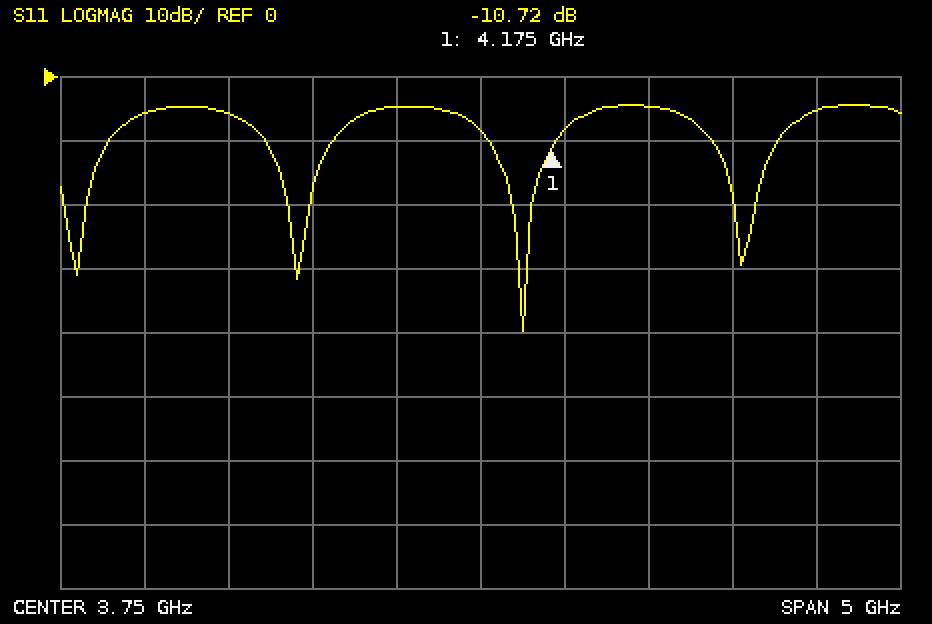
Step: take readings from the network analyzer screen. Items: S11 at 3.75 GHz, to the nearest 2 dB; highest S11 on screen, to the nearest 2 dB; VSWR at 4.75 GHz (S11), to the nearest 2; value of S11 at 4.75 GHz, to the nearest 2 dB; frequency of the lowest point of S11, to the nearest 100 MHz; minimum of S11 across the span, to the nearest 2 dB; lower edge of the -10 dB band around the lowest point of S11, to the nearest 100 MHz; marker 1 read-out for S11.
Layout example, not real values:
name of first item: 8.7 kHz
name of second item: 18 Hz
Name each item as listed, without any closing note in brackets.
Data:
S11 at 3.75 GHz, to the nearest 2 dB: -8 dB
highest S11 on screen, to the nearest 2 dB: -4 dB
VSWR at 4.75 GHz (S11), to the nearest 2: 4
value of S11 at 4.75 GHz, to the nearest 2 dB: -4 dB
frequency of the lowest point of S11, to the nearest 100 MHz: 4.0 GHz
minimum of S11 across the span, to the nearest 2 dB: -40 dB
lower edge of the -10 dB band around the lowest point of S11, to the nearest 100 MHz: 3.8 GHz
marker 1 read-out for S11: -10.72 dB
